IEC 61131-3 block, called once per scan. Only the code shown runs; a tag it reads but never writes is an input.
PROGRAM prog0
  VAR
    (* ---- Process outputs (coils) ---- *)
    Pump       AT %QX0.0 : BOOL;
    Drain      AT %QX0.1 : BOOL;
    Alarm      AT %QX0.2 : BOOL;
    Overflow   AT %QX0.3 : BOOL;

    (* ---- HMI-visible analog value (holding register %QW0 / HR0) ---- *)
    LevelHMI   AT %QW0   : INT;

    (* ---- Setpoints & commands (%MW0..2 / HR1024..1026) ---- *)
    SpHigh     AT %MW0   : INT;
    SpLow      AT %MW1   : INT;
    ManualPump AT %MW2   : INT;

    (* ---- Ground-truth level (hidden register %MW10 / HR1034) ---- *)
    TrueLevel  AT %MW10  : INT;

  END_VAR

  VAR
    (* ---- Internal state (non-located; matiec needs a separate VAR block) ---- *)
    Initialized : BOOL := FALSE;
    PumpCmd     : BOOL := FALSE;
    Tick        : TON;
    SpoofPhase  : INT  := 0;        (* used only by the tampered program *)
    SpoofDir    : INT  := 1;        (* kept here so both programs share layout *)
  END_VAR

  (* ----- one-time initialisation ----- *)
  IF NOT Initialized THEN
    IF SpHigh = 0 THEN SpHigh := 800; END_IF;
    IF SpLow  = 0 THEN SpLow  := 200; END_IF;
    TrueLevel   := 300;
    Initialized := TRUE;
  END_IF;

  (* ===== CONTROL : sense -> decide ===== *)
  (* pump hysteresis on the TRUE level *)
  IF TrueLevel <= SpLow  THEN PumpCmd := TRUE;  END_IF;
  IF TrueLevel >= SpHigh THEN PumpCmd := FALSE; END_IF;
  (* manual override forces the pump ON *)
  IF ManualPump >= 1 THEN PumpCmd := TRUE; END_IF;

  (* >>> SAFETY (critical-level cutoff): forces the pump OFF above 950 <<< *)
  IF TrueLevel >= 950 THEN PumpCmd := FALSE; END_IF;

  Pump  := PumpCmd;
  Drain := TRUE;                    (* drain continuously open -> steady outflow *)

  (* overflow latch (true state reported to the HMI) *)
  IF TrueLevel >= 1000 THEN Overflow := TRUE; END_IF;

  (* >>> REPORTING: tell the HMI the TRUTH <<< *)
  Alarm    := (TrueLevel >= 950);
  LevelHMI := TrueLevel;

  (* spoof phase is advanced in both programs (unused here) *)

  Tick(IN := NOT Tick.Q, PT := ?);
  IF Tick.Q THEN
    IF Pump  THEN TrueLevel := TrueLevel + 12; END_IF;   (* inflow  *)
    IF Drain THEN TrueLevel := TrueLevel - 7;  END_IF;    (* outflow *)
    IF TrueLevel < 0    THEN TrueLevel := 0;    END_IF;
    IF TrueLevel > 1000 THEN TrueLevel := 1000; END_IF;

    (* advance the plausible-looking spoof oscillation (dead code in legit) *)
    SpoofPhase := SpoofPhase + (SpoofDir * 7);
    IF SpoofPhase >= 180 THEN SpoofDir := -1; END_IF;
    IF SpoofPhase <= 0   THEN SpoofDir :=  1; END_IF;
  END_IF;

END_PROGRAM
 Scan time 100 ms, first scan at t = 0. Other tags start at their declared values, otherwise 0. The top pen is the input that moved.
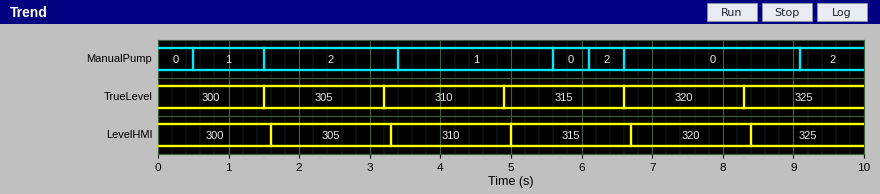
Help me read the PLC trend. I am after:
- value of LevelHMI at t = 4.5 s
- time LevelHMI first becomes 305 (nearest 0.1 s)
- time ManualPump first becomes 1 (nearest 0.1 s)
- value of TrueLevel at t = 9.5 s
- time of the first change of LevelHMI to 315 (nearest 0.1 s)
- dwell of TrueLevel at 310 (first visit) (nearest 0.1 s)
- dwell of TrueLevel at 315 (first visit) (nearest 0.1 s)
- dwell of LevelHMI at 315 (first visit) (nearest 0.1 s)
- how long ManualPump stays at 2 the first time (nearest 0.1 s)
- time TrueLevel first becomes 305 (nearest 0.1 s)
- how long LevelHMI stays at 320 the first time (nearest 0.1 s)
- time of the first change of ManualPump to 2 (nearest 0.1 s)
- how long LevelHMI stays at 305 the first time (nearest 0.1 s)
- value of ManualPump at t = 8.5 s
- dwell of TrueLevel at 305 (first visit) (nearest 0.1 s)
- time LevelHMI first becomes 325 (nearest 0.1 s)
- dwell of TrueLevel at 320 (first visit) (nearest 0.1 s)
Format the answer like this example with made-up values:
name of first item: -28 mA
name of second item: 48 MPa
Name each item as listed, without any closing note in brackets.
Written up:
value of LevelHMI at t = 4.5 s: 310
time LevelHMI first becomes 305: 1.6 s
time ManualPump first becomes 1: 0.5 s
value of TrueLevel at t = 9.5 s: 325
time of the first change of LevelHMI to 315: 5.0 s
dwell of TrueLevel at 310 (first visit): 1.7 s
dwell of TrueLevel at 315 (first visit): 1.7 s
dwell of LevelHMI at 315 (first visit): 1.7 s
how long ManualPump stays at 2 the first time: 1.9 s
time TrueLevel first becomes 305: 1.5 s
how long LevelHMI stays at 320 the first time: 1.7 s
time of the first change of ManualPump to 2: 1.5 s
how long LevelHMI stays at 305 the first time: 1.7 s
value of ManualPump at t = 8.5 s: 0
dwell of TrueLevel at 305 (first visit): 1.7 s
time LevelHMI first becomes 325: 8.4 s
dwell of TrueLevel at 320 (first visit): 1.7 s
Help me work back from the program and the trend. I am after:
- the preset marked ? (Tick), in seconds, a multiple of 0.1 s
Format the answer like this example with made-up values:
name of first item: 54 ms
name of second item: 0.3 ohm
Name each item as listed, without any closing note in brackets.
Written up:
the preset marked ? (Tick), in seconds, a multiple of 0.1 s: 1.5 s
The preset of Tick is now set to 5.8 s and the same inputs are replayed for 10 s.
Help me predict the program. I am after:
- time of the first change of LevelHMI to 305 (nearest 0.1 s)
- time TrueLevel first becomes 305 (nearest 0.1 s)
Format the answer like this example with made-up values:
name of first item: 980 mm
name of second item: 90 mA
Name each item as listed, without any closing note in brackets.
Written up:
time of the first change of LevelHMI to 305: 5.9 s
time TrueLevel first becomes 305: 5.8 s
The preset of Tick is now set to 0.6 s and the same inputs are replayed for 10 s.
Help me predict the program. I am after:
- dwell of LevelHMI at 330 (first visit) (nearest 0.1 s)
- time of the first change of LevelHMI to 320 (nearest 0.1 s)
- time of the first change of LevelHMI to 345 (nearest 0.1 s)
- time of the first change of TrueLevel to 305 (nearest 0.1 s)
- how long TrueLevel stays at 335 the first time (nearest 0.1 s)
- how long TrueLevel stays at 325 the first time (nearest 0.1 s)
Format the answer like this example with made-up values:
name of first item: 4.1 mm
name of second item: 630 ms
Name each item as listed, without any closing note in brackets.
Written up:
dwell of LevelHMI at 330 (first visit): 0.8 s
time of the first change of LevelHMI to 320: 3.1 s
time of the first change of LevelHMI to 345: 7.1 s
time of the first change of TrueLevel to 305: 0.6 s
how long TrueLevel stays at 335 the first time: 0.8 s
how long TrueLevel stays at 325 the first time: 0.8 s
